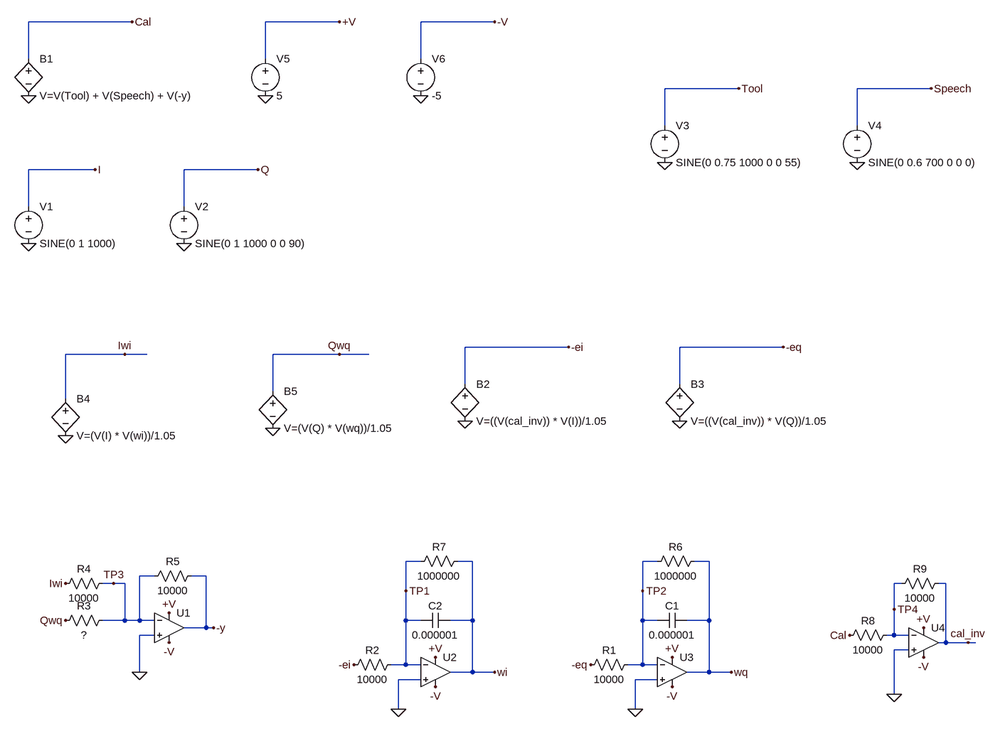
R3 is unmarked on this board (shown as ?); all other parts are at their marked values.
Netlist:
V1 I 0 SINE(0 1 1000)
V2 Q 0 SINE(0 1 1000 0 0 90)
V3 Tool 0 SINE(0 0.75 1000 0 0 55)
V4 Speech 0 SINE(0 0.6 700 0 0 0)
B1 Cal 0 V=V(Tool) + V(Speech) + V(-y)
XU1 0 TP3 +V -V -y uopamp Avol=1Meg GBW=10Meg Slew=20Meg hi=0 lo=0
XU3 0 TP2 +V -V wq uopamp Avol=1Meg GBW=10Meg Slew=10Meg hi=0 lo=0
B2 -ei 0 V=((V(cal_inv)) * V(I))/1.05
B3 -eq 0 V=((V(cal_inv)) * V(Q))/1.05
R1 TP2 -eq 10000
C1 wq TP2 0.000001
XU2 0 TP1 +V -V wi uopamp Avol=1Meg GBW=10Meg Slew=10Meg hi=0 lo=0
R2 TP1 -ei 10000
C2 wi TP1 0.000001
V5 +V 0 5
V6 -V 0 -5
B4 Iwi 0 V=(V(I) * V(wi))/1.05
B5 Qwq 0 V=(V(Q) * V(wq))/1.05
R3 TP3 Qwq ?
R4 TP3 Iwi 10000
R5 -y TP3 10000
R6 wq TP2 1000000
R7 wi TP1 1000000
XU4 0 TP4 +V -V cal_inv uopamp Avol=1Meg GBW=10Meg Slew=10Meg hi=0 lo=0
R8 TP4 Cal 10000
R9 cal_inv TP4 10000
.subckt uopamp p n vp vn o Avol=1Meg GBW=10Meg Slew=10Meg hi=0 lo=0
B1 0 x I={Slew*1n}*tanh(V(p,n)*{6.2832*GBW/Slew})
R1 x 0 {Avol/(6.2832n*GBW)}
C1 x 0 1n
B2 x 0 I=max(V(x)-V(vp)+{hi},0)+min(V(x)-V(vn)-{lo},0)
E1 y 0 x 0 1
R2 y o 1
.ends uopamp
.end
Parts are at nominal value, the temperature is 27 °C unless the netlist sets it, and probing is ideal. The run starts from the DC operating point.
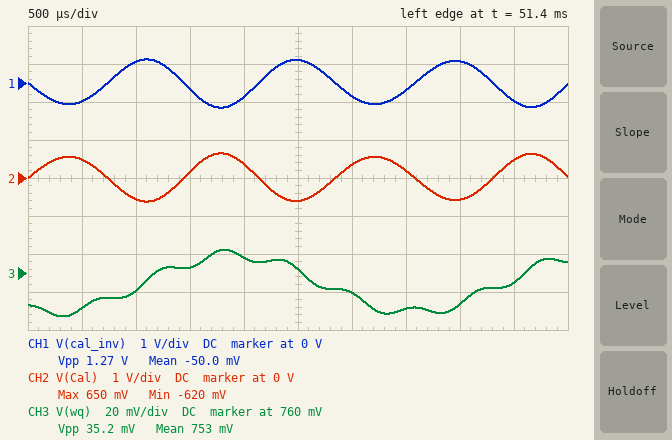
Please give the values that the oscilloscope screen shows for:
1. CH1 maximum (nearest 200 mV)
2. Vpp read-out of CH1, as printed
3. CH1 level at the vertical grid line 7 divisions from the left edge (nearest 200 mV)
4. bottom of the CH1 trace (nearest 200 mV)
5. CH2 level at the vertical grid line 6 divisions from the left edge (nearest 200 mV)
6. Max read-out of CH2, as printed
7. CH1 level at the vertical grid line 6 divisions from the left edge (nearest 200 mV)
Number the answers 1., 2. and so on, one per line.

1. 600 mV
2. 1.27 V
3. -200 mV
4. -600 mV
5. 400 mV
6. 650 mV
7. -400 mV
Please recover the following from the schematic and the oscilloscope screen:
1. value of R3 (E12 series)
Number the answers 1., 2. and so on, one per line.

1. 12 kΩ
